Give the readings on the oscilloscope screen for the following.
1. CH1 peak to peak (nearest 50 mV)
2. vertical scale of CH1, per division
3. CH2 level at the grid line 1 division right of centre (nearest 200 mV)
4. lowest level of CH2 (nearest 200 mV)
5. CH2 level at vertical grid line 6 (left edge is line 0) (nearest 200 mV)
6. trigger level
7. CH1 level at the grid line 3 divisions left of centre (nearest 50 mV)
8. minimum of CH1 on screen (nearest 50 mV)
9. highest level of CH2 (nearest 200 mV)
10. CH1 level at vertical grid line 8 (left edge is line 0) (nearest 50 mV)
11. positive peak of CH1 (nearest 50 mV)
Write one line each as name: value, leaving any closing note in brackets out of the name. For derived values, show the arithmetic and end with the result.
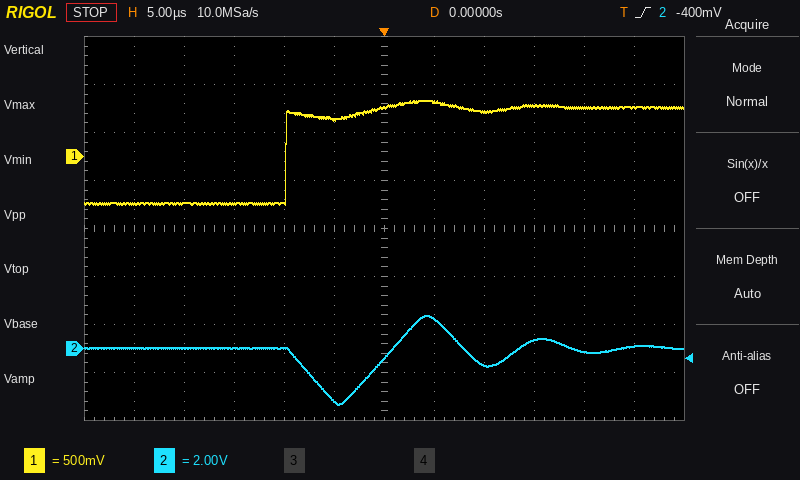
CH1 peak to peak: 600 mV − (-500 mV) = 1.10 V
vertical scale of CH1, per division: 500 mV
CH2 level at the grid line 1 division right of centre: 1.2 V
lowest level of CH2: -2.4 V
CH2 level at vertical grid line 6 (left edge is line 0): -400 mV
trigger level: -400 mV
CH1 level at the grid line 3 divisions left of centre: -500 mV
minimum of CH1 on screen: -500 mV
highest level of CH2: 1.4 V
CH1 level at vertical grid line 8 (left edge is line 0): 450 mV
positive peak of CH1: 600 mV
